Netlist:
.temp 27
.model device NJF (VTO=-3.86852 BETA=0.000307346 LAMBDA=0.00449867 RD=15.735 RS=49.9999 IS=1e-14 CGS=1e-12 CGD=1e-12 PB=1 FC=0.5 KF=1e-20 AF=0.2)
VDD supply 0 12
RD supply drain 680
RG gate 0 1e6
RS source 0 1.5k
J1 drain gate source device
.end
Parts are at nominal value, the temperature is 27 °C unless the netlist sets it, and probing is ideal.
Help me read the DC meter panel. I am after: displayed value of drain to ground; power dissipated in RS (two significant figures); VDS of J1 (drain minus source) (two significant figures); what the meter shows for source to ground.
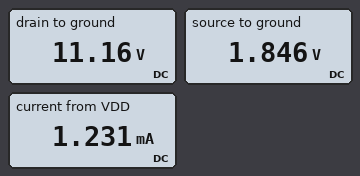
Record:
11.16 V
2.3 mW
9.3 V
1.846 V
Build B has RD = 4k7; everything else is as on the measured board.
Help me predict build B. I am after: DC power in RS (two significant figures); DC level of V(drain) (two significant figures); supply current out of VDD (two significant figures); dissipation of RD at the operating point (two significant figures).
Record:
2.2 mW
6.3 V
1.2 mA
7.0 mW
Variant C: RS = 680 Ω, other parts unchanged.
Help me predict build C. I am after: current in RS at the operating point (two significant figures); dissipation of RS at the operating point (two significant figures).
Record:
1.9 mA
2.5 mW
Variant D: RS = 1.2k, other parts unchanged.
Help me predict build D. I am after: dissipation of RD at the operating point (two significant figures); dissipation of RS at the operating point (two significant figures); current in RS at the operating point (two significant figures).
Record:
1.4 mW
2.4 mW
1.4 mA
